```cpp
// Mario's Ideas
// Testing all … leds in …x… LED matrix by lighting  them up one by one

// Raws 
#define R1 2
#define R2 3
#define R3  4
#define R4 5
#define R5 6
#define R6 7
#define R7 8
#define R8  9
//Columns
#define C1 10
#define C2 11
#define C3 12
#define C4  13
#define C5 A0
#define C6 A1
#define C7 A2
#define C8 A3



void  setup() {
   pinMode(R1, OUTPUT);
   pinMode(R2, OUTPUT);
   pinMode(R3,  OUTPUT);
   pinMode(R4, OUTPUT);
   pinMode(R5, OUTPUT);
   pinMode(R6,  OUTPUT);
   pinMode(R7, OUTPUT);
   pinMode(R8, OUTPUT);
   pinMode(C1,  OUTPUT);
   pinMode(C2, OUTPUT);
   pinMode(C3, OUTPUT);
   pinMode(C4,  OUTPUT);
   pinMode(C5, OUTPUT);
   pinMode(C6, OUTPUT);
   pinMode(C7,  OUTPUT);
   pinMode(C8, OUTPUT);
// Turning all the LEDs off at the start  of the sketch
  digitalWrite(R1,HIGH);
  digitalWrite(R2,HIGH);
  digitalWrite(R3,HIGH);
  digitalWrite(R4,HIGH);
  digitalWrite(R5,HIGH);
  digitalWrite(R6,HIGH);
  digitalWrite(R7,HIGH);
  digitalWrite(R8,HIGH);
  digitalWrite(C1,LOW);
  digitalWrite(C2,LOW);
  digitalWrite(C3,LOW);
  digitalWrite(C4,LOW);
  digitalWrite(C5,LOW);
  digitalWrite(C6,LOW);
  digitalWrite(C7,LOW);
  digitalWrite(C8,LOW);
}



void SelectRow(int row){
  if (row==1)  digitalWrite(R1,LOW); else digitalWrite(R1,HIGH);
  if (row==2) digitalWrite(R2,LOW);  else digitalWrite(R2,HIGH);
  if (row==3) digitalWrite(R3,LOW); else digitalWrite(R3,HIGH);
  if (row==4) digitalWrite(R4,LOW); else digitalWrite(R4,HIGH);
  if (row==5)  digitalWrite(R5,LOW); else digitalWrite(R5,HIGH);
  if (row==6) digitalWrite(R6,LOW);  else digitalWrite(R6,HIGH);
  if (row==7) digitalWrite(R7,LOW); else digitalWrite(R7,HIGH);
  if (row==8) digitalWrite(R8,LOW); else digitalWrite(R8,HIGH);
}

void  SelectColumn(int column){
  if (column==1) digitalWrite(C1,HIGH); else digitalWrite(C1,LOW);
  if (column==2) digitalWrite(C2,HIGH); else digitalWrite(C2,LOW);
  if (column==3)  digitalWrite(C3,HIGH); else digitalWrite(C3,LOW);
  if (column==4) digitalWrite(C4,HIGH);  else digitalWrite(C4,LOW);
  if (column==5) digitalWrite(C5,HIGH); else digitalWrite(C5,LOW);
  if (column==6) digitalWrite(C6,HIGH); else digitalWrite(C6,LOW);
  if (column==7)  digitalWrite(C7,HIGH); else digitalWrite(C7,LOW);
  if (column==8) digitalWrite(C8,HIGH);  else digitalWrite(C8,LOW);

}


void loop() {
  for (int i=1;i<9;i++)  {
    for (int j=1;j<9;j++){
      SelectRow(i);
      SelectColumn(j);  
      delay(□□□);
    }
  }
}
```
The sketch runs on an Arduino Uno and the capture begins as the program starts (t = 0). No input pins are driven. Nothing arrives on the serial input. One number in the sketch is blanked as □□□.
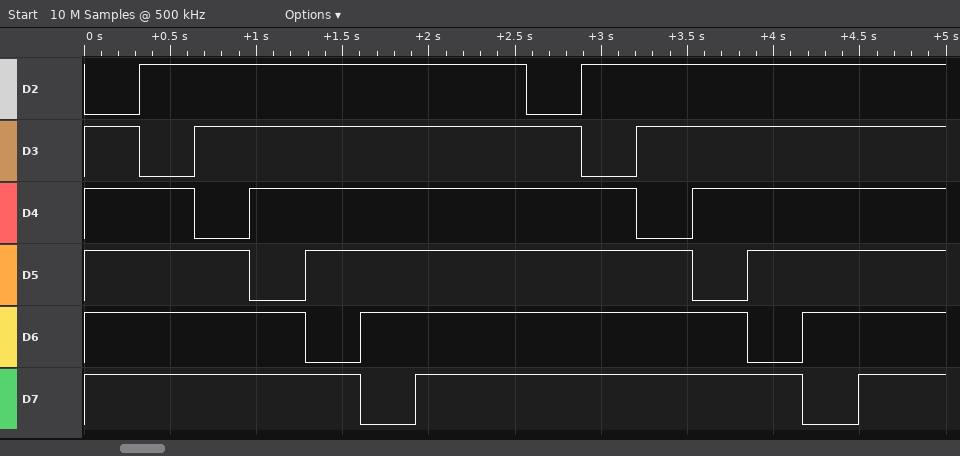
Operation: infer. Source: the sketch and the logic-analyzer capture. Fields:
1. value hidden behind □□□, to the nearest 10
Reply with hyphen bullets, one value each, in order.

- 40
